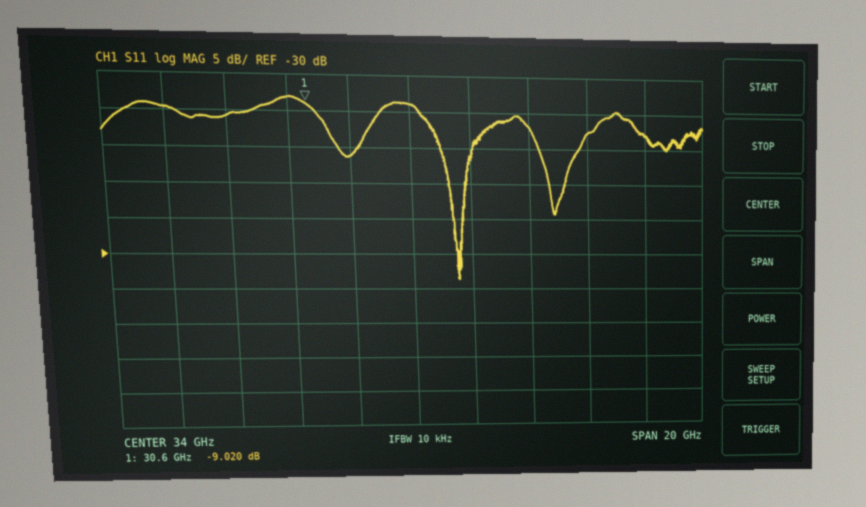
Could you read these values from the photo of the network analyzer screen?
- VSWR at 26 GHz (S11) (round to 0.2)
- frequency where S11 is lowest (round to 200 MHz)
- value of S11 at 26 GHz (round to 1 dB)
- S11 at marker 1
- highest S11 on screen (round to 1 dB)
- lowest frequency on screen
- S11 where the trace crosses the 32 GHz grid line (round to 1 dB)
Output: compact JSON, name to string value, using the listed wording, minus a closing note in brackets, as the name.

{"VSWR at 26 GHz (S11)": "2.0", "frequency where S11 is lowest": "35.6 GHz", "value of S11 at 26 GHz": "-10 dB", "S11 at marker 1": "-9.020 dB", "highest S11 on screen": "-8 dB", "lowest frequency on screen": "24 GHz", "S11 where the trace crosses the 32 GHz grid line": "-16 dB"}
